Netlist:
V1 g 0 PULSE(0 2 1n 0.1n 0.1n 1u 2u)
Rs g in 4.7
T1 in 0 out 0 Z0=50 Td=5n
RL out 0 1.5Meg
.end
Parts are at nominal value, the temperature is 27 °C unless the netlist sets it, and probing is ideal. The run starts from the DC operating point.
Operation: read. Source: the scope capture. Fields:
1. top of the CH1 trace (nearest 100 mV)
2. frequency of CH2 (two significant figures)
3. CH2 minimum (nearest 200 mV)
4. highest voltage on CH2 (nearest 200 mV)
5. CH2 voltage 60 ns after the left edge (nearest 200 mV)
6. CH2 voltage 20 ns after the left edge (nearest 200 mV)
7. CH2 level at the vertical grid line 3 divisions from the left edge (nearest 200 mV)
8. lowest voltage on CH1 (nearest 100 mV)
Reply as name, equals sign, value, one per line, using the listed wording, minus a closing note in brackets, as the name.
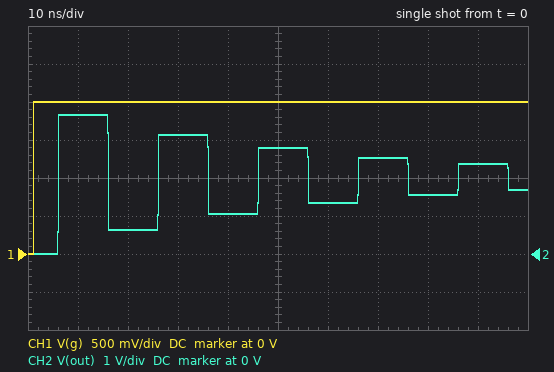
top of the CH1 trace = 2.0 V
frequency of CH2 = 50 MHz
CH2 minimum = 0 V
highest voltage on CH2 = 3.6 V
CH2 voltage 60 ns after the left edge = 1.4 V
CH2 voltage 20 ns after the left edge = 600 mV
CH2 level at the vertical grid line 3 divisions from the left edge = 3.2 V
lowest voltage on CH1 = 0 V
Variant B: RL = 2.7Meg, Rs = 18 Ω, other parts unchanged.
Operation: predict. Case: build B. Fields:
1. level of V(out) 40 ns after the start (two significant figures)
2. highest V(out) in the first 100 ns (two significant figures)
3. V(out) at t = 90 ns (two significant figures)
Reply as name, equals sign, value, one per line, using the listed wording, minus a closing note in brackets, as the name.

level of V(out) 40 ns after the start = 1.9 V
highest V(out) in the first 100 ns = 2.9 V
V(out) at t = 90 ns = 2.0 V
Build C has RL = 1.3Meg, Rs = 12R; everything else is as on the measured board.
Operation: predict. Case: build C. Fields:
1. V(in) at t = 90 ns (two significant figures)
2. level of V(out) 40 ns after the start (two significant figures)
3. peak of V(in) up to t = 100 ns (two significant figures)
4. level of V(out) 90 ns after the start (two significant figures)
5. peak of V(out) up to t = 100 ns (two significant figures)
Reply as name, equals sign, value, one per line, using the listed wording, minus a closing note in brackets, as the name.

V(in) at t = 90 ns = 2.0 V
level of V(out) 40 ns after the start = 1.7 V
peak of V(in) up to t = 100 ns = 2.2 V
level of V(out) 90 ns after the start = 2.0 V
peak of V(out) up to t = 100 ns = 3.2 V
